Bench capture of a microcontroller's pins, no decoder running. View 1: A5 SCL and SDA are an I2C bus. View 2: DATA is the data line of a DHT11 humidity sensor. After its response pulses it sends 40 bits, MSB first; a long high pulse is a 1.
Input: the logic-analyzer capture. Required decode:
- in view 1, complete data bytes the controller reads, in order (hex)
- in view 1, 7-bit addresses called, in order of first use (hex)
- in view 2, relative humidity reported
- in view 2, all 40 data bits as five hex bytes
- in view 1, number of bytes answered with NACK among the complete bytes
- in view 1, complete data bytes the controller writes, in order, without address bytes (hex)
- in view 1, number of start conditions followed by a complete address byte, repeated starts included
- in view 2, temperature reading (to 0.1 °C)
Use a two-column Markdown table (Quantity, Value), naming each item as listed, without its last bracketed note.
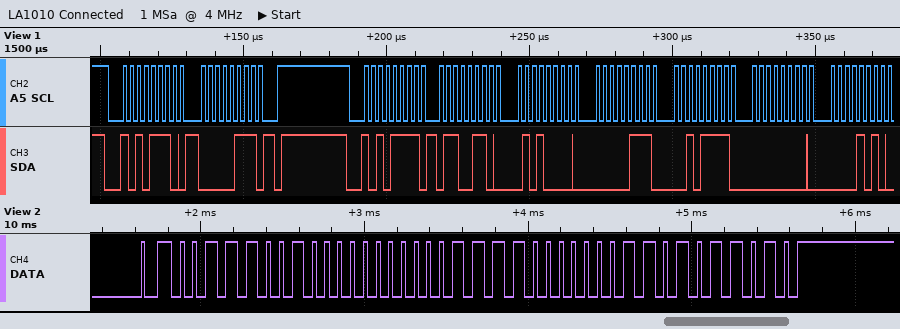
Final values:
| Quantity | Value |
|---|---|
| in view 1, complete data bytes the controller reads, in order | 66 50 07 2F 00 0A |
| in view 1, 7-bit addresses called, in order of first use | 0x57 |
| in view 2, relative humidity reported | 57 % |
| in view 2, all 40 data bits as five hex bytes | 39 00 1E 03 5A |
| in view 1, number of bytes answered with NACK among the complete bytes | 0 |
| in view 1, complete data bytes the controller writes, in order, without address bytes | 07 |
| in view 1, number of start conditions followed by a complete address byte, repeated starts included | 2 |
| in view 2, temperature reading | 30.3 °C |
